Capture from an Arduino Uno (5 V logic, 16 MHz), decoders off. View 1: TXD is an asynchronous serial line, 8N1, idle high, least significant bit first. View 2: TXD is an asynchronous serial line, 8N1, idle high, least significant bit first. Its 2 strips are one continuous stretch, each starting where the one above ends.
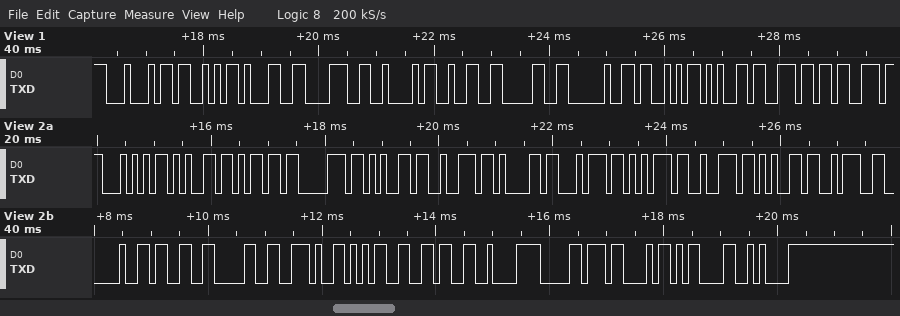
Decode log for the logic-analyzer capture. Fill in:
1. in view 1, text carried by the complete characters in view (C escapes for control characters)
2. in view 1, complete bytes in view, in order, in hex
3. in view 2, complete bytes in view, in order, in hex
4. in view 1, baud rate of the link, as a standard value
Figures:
"DS18B20 Sens"
0x44 0x53 0x31 0x38 0x42 0x32 0x30 0x20 0x53 0x65 0x6E 0x73
54 65 6D 70 65 72 61 74 75 72 65 3A 20 33 30 2E 35 36 C2 B0 43 0D 0A
9600 baud
